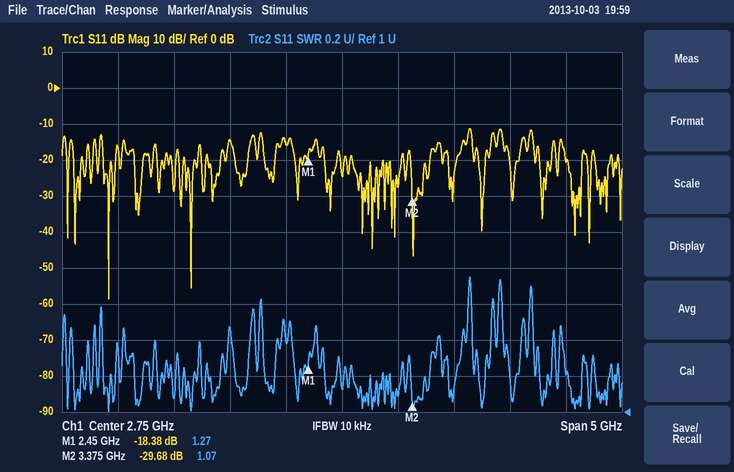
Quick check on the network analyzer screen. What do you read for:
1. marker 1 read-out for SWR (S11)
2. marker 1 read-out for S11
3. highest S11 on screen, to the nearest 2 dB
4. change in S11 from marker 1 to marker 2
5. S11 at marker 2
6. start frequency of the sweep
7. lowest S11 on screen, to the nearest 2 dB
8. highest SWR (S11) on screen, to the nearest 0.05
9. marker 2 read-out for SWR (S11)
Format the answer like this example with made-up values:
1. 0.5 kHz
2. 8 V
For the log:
1. 1.27
2. -18.38 dB
3. -12 dB
4. -11.30 dB
5. -29.68 dB
6. 250 MHz
7. -58 dB
8. 1.75
9. 1.07
